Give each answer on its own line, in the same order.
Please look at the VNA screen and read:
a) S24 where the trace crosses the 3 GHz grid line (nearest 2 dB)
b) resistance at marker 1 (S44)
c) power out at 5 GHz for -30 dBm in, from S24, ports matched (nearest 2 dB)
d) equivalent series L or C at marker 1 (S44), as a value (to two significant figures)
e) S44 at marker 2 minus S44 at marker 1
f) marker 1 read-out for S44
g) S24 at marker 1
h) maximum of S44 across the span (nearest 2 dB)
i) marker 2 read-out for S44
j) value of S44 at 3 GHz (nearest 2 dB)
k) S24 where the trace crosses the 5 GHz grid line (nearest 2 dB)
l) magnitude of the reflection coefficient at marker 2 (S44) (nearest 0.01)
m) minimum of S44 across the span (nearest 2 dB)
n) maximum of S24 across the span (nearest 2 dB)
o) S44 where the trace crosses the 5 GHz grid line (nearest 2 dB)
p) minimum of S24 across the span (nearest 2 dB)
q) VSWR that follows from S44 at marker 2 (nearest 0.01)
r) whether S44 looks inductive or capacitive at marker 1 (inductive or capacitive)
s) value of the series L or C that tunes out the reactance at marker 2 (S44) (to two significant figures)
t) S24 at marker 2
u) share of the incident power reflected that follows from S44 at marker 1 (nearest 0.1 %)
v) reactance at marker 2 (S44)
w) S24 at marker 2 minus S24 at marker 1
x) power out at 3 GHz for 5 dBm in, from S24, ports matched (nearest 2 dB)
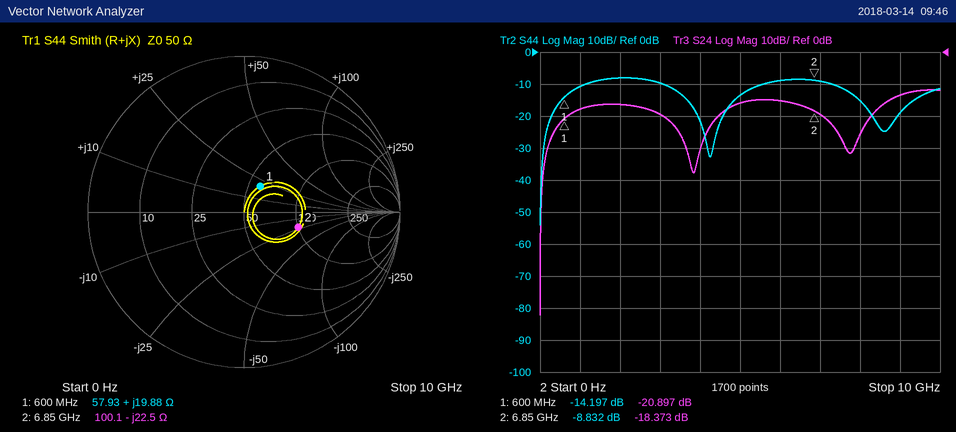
-20 dB
57.93 Ω
-46 dBm
5.3 nH
5.365 dB
-14.197 dB
-20.897 dB
-8 dB
-8.832 dB
-10 dB
-16 dB
0.36
-54 dB
-12 dB
-14 dB
-82 dB
2.13
inductive
520 pH
-18.373 dB
3.8 %
-22.5 Ω
2.524 dB
-14 dBm
